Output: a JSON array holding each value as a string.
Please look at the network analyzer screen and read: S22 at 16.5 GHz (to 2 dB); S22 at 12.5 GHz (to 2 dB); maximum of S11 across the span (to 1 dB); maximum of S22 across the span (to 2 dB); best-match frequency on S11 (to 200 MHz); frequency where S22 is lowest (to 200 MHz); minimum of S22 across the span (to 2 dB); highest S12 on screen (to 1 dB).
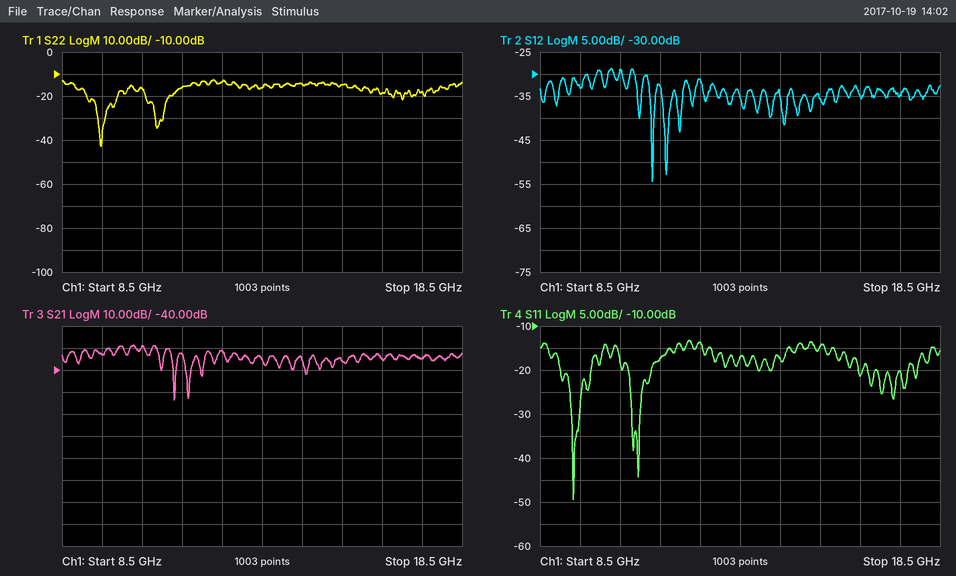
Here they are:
["-18 dB", "-14 dB", "-13 dB", "-12 dB", "9.4 GHz", "9.4 GHz", "-42 dB", "-29 dB"]
